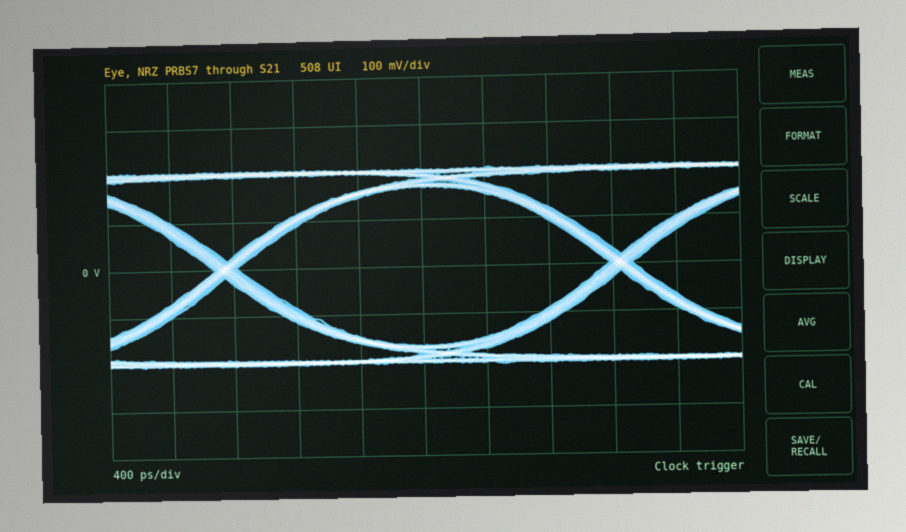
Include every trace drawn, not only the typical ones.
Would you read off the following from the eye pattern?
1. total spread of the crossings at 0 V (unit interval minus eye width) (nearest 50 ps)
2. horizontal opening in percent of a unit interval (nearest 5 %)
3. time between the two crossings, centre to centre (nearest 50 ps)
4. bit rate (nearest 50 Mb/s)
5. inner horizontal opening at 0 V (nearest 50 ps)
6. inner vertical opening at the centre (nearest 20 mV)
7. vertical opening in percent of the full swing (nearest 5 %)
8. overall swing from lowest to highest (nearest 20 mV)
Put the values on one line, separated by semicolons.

150 ps; 95 %; 2.50 ns; 400 Mb/s; 2.35 ns; 340 mV; 80 %; 420 mV
